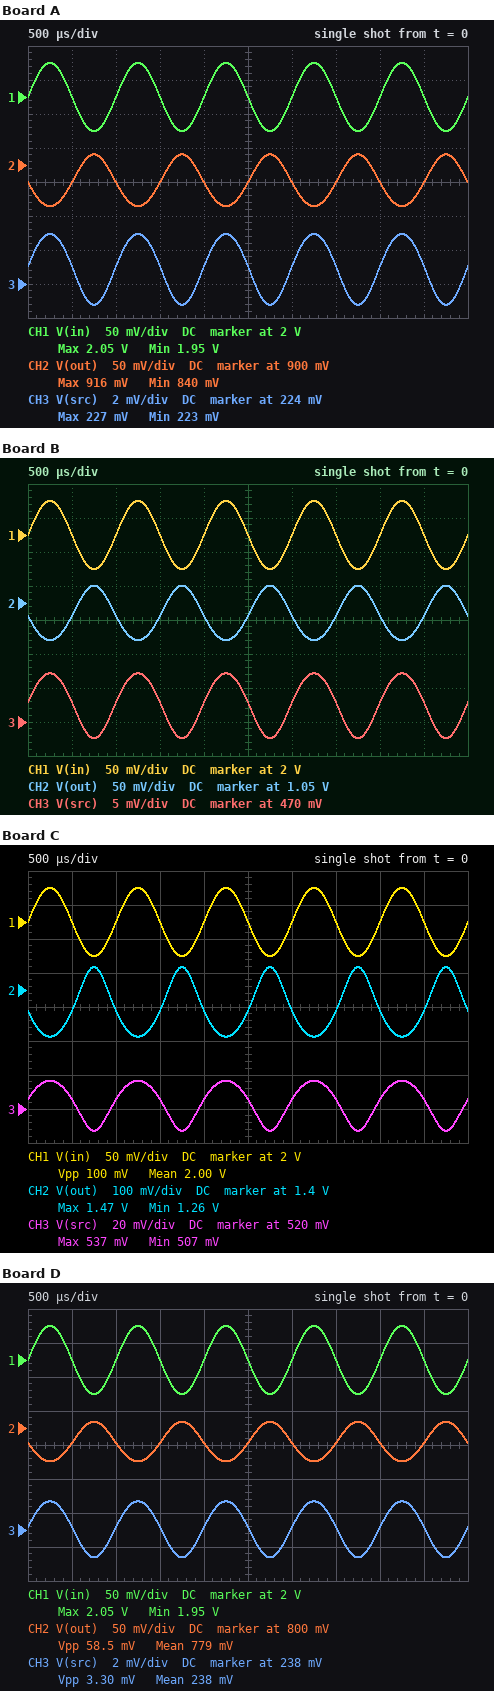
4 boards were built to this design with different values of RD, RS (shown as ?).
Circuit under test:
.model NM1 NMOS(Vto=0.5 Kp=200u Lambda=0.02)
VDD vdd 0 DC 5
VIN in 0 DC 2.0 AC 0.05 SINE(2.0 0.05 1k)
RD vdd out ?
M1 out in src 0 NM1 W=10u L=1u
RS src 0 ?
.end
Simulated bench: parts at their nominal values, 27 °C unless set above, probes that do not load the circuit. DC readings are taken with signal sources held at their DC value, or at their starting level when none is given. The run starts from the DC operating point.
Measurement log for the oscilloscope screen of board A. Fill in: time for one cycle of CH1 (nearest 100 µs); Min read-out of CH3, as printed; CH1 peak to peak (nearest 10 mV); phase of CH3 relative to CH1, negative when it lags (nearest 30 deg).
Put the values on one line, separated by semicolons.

1.0 ms; 223 mV; 100 mV; 0 deg
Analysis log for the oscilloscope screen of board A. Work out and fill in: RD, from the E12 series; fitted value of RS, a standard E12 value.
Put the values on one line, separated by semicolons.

3.3 kΩ; 180 Ω
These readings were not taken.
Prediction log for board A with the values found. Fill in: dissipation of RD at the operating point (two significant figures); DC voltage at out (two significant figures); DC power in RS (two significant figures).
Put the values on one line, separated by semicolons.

5.2 mW; 870 mV; 280 µW
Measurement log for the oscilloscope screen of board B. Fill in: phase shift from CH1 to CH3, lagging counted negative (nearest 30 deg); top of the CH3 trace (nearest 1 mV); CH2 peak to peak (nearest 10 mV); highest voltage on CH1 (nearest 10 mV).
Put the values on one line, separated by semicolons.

0 deg; 477 mV; 80 mV; 2.05 V
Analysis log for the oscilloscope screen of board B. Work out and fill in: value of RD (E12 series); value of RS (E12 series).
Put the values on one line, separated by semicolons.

4.7 kΩ; 560 Ω
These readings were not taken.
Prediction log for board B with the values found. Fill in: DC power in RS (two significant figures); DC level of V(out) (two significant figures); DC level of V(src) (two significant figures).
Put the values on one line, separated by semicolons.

400 µW; 1.0 V; 470 mV
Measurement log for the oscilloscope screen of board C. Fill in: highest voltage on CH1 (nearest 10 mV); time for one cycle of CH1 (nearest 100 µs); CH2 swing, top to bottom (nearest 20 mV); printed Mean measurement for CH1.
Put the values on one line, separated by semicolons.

2.05 V; 1.0 ms; 200 mV; 2.00 V
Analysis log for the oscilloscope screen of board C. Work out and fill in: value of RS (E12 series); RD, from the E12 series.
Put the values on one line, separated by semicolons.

560 Ω; 3.9 kΩ
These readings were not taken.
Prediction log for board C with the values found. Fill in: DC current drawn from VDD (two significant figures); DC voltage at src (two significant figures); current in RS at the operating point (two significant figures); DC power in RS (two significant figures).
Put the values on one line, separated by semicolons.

940 µA; 530 mV; 940 µA; 490 µW
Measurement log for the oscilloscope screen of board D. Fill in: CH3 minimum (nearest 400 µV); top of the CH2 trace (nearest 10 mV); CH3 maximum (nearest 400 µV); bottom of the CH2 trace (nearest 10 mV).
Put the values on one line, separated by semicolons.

236.4 mV; 810 mV; 239.6 mV; 750 mV
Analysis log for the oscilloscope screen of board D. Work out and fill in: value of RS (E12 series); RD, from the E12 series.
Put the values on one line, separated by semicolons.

220 Ω; 3.9 kΩ
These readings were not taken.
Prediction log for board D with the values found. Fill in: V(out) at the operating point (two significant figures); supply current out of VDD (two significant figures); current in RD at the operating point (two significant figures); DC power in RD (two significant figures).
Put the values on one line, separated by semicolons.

780 mV; 1.1 mA; 1.1 mA; 4.6 mW
